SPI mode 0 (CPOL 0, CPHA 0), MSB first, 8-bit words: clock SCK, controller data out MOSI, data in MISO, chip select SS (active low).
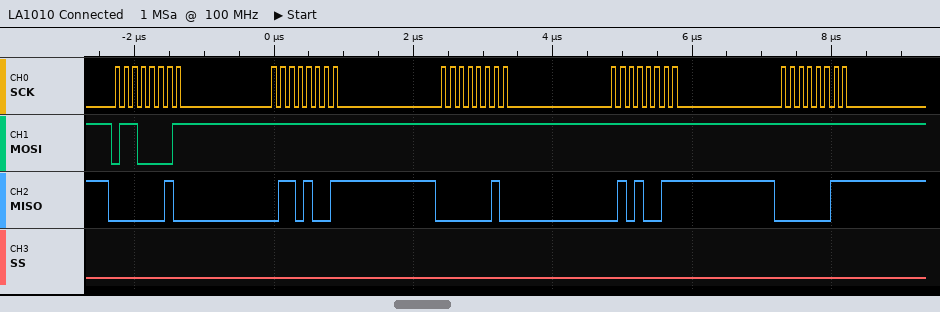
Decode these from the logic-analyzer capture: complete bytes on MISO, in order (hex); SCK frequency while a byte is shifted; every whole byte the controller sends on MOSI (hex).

02 69 02 53 03
8 MHz
61 FF FF FF FF
